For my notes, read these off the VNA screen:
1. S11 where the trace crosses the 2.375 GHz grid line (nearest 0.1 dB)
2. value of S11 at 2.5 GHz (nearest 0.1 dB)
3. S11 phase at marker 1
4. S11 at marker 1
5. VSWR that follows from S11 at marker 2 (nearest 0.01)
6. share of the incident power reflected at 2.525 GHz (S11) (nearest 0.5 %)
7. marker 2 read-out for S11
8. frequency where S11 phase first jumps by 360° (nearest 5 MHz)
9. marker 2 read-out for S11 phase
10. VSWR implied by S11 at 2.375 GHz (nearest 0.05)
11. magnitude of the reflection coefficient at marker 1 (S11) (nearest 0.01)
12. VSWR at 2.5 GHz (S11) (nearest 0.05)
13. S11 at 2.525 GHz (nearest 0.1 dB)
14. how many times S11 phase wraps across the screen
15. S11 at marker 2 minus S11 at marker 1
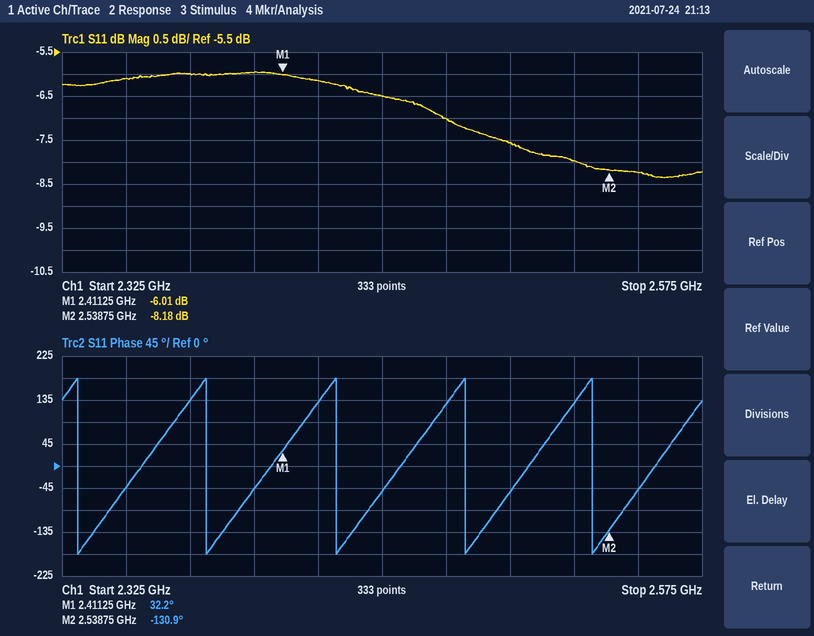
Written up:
-6.0 dB
-7.6 dB
32.2°
-6.01 dB
2.28
16.0 %
-8.18 dB
2.330 GHz
-130.9°
3.00
0.50
2.45
-8.0 dB
5
-2.17 dB
